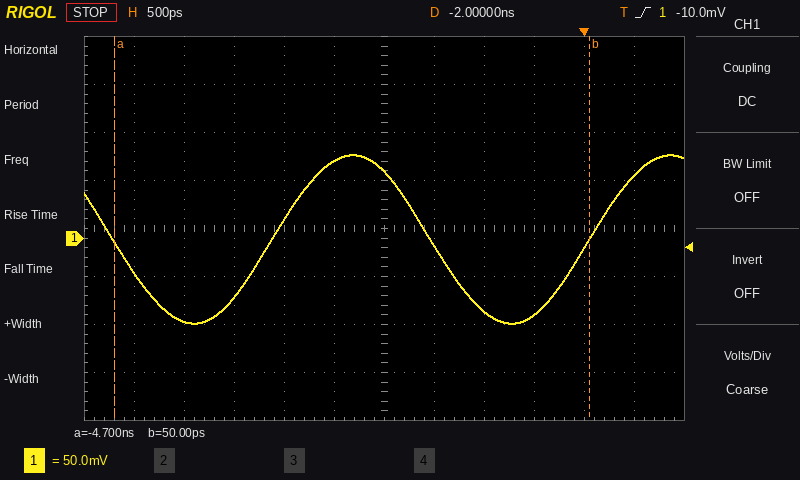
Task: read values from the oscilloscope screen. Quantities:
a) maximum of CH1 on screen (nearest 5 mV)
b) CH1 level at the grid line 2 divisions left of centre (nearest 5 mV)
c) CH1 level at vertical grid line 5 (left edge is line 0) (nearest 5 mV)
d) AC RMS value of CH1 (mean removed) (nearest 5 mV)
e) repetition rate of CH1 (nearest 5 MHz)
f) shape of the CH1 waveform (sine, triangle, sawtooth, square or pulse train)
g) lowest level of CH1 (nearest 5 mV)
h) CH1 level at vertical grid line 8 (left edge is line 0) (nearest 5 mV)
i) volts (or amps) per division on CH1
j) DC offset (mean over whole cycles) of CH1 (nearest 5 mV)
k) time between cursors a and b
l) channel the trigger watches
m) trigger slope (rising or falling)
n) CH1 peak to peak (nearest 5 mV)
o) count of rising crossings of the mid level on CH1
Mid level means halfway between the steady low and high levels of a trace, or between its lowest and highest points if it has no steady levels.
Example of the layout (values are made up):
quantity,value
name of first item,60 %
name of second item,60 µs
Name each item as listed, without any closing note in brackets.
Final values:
quantity,value
maximum of CH1 on screen,85 mV
CH1 level at the grid line 2 divisions left of centre,20 mV
CH1 level at vertical grid line 5 (left edge is line 0),80 mV
AC RMS value of CH1 (mean removed),60 mV
repetition rate of CH1,315 MHz
shape of the CH1 waveform,sine
lowest level of CH1,-90 mV
CH1 level at vertical grid line 8 (left edge is line 0),-75 mV
volts (or amps) per division on CH1,50 mV
DC offset (mean over whole cycles) of CH1,0 mV
time between cursors a and b,4.75 ns
channel the trigger watches,CH1
trigger slope,rising
CH1 peak to peak,175 mV
count of rising crossings of the mid level on CH1,2
